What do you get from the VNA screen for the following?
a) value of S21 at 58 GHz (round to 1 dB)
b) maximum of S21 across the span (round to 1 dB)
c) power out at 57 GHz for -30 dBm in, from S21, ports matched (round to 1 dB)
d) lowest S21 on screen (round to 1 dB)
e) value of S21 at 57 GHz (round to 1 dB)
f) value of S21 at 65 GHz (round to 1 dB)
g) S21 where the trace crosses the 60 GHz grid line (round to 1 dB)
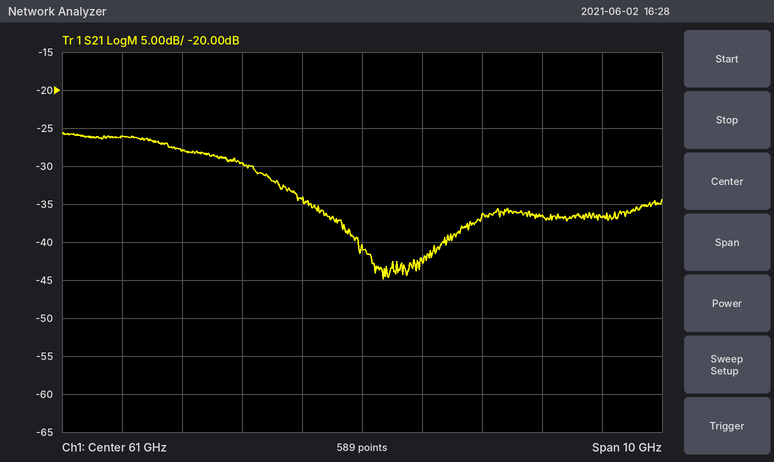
-28 dB
-26 dB
-56 dBm
-45 dB
-26 dB
-37 dB
-34 dB
